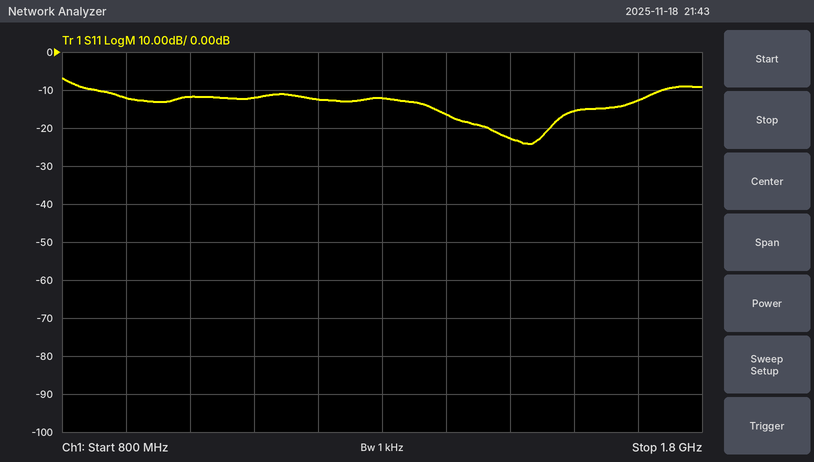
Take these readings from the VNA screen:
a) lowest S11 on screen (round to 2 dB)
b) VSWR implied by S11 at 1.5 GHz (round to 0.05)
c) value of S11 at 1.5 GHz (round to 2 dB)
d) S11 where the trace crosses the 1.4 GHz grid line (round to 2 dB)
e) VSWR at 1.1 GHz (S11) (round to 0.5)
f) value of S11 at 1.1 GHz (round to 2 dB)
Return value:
-24 dB
1.15
-22 dB
-16 dB
1.5
-12 dB
